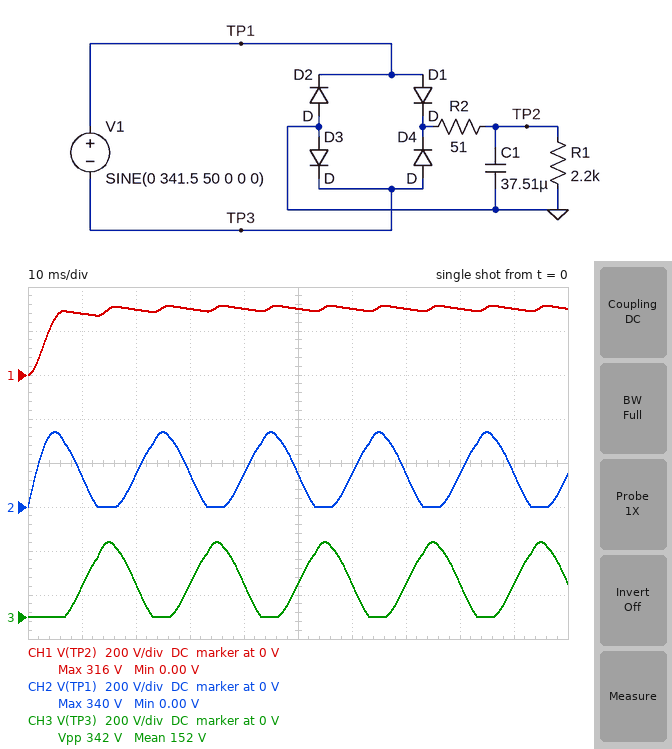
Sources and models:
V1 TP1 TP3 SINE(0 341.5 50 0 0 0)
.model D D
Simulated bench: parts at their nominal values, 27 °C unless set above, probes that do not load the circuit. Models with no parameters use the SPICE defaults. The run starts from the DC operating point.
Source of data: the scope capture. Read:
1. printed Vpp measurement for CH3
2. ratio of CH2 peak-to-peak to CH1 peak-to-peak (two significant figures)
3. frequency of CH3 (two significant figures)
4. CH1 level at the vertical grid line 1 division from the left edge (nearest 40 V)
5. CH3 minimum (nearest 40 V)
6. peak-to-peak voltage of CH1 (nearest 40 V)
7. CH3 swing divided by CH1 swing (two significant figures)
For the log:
342 V
1.1
50 Hz
280 V
0 V
320 V
1.1
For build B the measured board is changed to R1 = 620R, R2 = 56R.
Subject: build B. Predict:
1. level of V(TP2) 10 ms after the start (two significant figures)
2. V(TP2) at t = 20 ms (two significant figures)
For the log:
240 V
250 V
